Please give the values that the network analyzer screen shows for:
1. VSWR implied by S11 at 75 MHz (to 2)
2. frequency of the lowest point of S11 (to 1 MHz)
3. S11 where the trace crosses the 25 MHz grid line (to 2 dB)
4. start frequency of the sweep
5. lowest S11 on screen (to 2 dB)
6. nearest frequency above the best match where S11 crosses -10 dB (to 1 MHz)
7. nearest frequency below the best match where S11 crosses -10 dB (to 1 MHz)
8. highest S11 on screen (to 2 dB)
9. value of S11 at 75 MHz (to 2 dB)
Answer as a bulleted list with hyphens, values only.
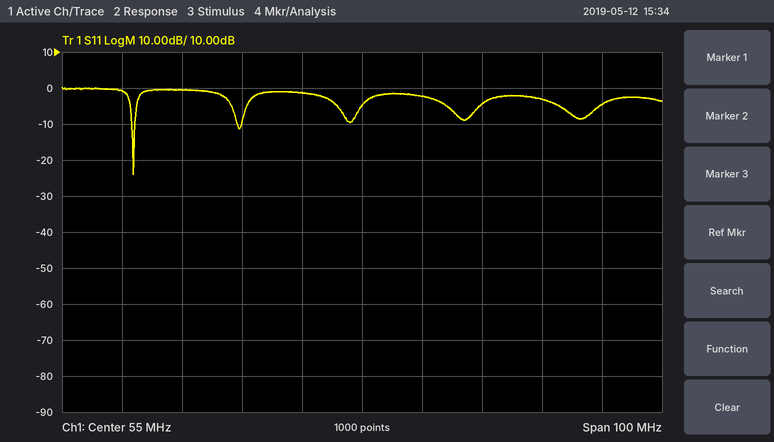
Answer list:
- 4
- 17 MHz
- 0 dB
- 5 MHz
- -24 dB
- 17 MHz
- 17 MHz
- 0 dB
- -4 dB
